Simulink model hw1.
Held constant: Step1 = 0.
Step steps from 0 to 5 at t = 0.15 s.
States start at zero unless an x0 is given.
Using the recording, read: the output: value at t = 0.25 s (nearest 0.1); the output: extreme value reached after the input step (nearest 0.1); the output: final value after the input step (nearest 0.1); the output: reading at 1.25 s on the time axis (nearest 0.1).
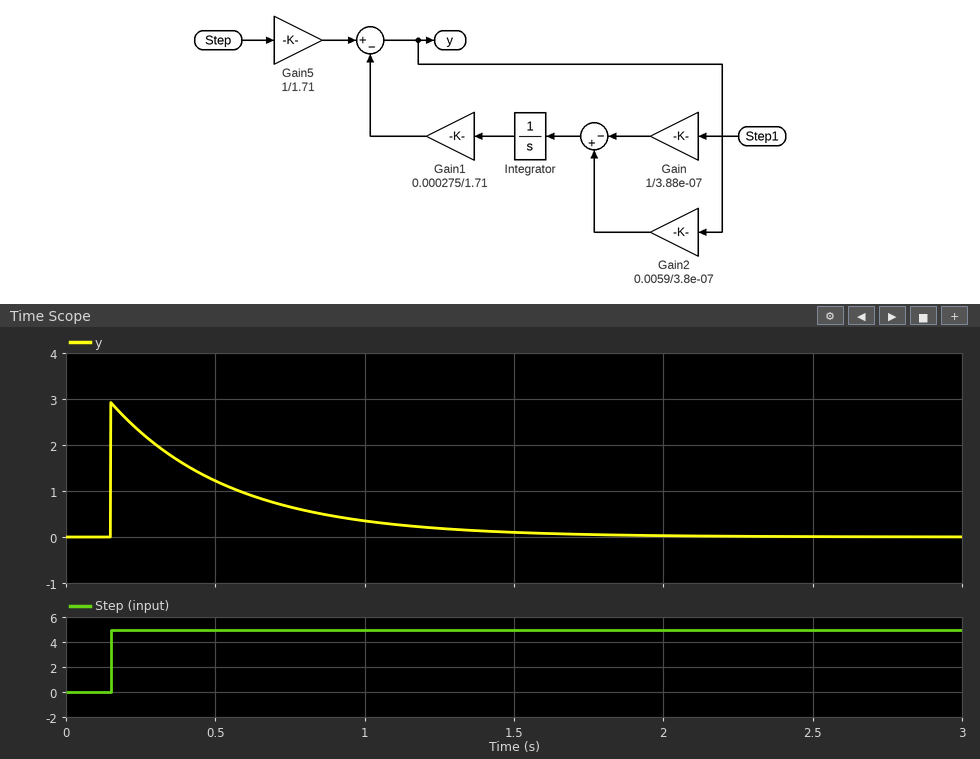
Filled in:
2.3
2.9
0.0
0.2
